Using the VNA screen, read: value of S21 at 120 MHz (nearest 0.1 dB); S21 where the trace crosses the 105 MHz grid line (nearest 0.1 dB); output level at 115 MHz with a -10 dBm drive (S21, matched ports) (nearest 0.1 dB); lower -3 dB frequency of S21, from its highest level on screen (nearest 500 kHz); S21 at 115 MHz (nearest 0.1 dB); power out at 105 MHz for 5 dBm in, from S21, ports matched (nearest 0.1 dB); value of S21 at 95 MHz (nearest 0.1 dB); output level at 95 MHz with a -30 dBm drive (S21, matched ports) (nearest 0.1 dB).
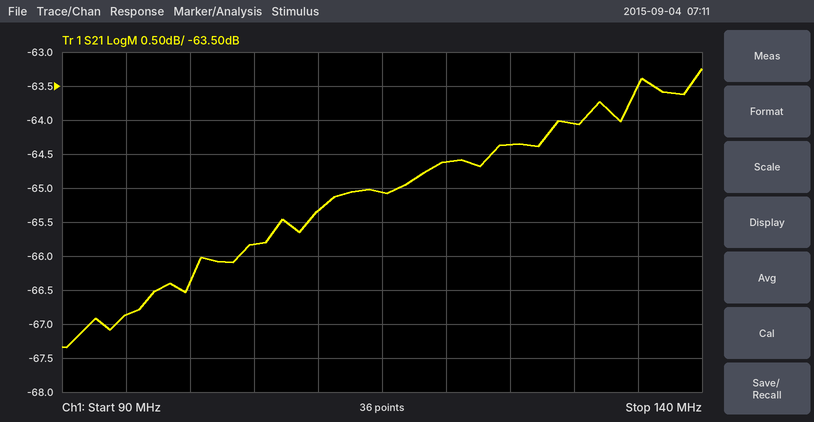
-64.6 dB
-65.8 dB
-75.1 dBm
100.5 MHz
-65.1 dB
-60.8 dBm
-66.9 dB
-96.9 dBm
